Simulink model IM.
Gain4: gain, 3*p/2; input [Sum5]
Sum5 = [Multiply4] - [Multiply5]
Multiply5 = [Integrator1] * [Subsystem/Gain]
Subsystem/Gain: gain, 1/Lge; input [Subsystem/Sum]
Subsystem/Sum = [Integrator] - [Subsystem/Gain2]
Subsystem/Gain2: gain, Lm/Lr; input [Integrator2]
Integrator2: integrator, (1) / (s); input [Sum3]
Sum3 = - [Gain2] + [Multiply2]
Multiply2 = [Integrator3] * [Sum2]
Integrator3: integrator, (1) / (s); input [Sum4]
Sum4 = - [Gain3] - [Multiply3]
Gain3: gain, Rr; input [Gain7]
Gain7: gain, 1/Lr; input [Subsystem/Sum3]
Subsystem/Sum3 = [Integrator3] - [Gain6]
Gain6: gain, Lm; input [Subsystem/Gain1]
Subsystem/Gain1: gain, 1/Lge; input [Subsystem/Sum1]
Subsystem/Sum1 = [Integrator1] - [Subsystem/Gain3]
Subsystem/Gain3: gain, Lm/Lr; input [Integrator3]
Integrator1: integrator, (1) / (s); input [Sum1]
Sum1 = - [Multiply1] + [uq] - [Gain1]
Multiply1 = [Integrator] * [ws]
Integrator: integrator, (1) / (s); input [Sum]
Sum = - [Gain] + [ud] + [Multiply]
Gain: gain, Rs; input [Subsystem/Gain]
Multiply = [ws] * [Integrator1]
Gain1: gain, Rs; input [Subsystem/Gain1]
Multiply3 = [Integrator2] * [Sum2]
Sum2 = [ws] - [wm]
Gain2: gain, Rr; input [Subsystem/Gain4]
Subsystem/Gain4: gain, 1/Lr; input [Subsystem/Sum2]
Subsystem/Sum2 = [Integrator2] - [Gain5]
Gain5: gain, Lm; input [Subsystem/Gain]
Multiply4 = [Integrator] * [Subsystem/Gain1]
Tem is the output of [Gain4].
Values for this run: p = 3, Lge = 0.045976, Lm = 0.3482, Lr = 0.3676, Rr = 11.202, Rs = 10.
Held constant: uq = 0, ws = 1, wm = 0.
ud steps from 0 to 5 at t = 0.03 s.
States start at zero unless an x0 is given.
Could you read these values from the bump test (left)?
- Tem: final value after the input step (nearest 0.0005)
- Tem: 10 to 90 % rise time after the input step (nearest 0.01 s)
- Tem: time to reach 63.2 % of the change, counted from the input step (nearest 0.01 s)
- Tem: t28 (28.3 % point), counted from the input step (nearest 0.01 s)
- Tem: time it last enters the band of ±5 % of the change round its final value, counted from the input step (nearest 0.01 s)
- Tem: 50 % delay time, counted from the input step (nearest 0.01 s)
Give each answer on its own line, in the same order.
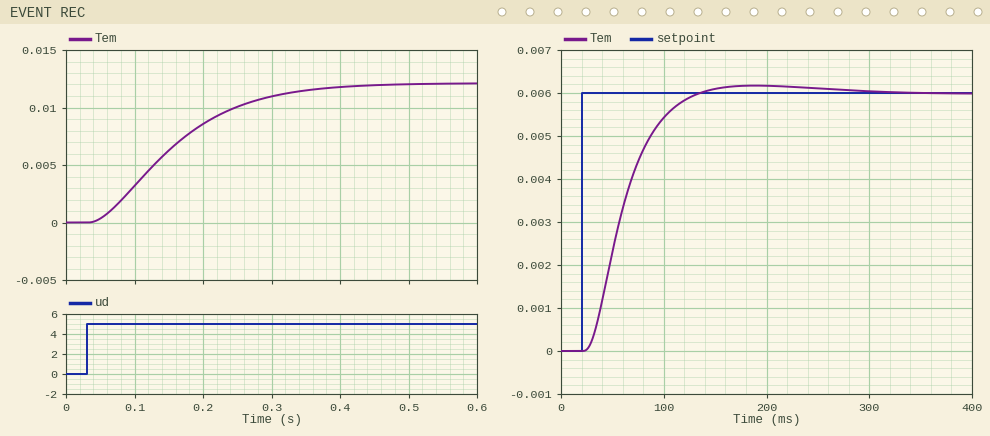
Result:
0.0120
0.23 s
0.15 s
0.07 s
0.32 s
0.12 s
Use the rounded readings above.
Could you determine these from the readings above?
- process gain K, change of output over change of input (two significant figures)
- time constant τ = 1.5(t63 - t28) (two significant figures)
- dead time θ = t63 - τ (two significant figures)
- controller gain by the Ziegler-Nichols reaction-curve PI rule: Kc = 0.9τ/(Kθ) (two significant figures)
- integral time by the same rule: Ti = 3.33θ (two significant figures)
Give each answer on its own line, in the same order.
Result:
0.0024
0.12 s
0.030 s
1500
0.100 s
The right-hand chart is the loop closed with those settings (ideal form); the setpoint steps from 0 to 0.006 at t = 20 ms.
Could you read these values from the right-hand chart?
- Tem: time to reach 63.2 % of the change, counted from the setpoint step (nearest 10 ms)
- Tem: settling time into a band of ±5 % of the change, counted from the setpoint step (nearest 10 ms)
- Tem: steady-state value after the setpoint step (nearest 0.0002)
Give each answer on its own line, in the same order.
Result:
50 ms
90 ms
0.0060
